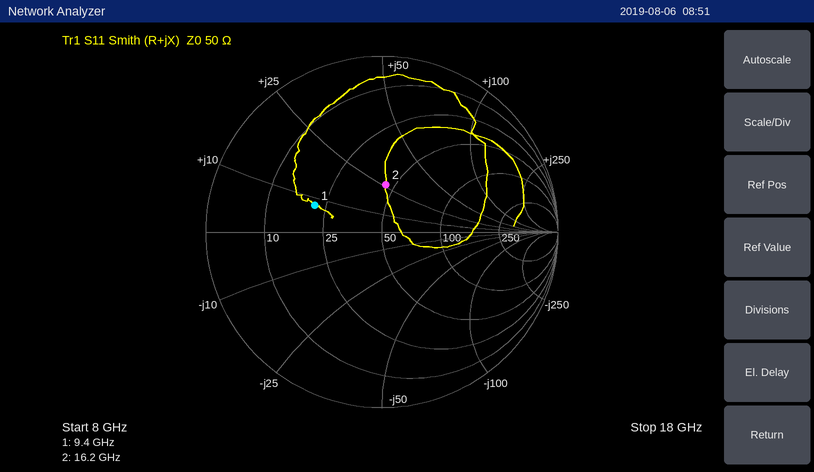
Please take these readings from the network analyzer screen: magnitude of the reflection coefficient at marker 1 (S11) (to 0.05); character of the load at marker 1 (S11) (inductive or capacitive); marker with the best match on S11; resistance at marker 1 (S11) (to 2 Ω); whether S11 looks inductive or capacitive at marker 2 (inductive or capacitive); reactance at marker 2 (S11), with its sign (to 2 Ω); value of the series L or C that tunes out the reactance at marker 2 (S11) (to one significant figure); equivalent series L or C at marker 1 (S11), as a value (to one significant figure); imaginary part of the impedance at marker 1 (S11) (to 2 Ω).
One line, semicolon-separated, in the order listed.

0.40; inductive; marker 2; 22 Ω; inductive; +26 Ω; 400 fF; 100 pH; +8 Ω
